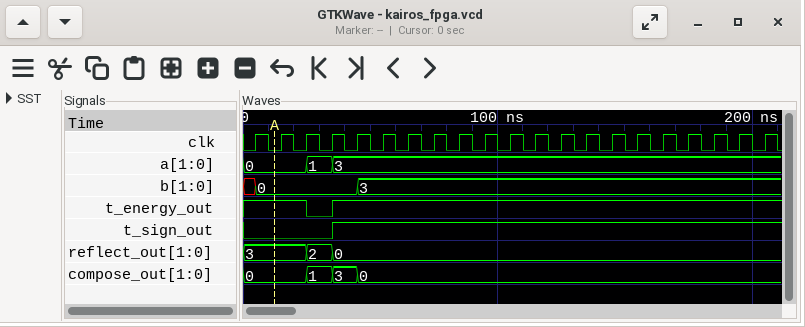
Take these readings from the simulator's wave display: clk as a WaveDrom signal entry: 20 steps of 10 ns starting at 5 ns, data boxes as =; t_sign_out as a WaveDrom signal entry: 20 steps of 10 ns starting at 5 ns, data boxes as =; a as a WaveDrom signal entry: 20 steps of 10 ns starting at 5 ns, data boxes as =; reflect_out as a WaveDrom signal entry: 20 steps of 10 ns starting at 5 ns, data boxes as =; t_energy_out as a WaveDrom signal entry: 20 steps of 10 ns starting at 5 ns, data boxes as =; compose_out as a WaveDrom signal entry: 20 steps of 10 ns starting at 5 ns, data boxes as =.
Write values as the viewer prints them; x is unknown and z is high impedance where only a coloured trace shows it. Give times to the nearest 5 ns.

{name: 'clk', wave: 'p...................'}
{name: 't_sign_out', wave: '0..1................'}
{name: 'a', wave: '=.==................', data: '0 1 3'}
{name: 'reflect_out', wave: '=.==................', data: '3 2 0'}
{name: 't_energy_out', wave: '1.01................'}
{name: 'compose_out', wave: '=.===...............', data: '0 1 3 0'}
